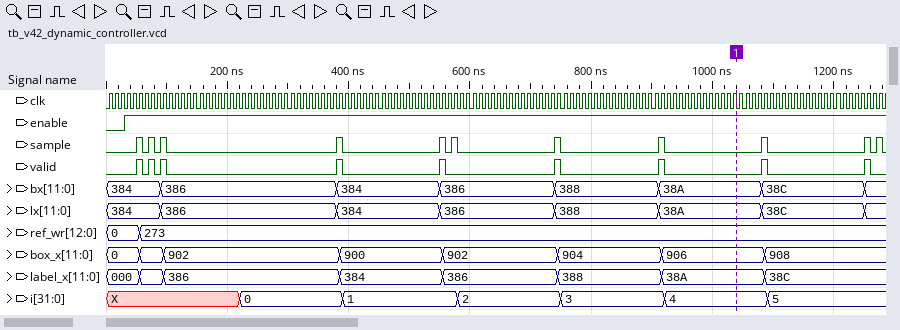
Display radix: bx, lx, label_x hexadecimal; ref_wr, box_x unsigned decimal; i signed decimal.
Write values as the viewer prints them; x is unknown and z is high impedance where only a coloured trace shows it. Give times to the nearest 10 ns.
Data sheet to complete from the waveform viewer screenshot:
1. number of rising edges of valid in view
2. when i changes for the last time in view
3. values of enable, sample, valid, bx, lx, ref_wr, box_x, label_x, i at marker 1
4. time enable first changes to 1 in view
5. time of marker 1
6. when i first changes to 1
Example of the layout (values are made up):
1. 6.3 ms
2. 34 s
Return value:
1. 9
2. 1090 ns
3. enable=1, sample=0, valid=0, bx=38A, lx=38A, ref_wr=273, box_x=906, label_x=38A, i=4
4. 30 ns
5. 1040 ns
6. 390 ns
